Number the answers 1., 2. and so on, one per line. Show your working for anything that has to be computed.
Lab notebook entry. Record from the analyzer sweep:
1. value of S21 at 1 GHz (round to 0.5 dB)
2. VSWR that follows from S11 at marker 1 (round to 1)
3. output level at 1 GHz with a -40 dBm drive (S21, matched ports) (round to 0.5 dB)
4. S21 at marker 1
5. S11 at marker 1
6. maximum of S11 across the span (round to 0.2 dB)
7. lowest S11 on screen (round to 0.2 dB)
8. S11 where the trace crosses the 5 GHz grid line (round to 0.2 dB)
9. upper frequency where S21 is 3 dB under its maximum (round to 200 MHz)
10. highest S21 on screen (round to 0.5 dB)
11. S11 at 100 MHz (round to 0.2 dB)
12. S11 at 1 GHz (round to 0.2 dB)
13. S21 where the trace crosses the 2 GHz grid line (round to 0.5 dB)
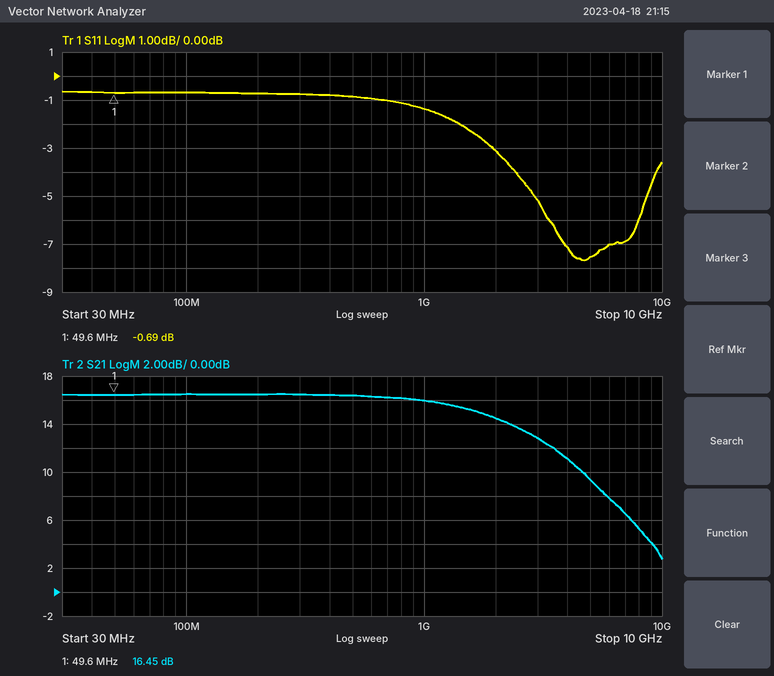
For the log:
1. 16.0 dB
2. (1 + 0.9236)/(1 − 0.9236) ≈ 25
3. -40 dBm + (16.0 dB) = -24.0 dBm
4. 16.45 dB
5. -0.69 dB
6. -0.6 dB
7. -7.6 dB
8. -7.6 dB
9. 2.6 GHz
10. 16.5 dB
11. -0.6 dB
12. -1.4 dB
13. 14.5 dB
